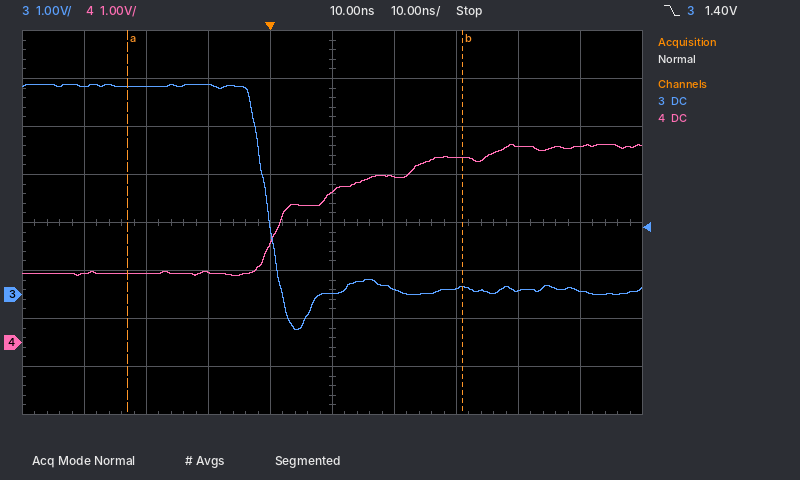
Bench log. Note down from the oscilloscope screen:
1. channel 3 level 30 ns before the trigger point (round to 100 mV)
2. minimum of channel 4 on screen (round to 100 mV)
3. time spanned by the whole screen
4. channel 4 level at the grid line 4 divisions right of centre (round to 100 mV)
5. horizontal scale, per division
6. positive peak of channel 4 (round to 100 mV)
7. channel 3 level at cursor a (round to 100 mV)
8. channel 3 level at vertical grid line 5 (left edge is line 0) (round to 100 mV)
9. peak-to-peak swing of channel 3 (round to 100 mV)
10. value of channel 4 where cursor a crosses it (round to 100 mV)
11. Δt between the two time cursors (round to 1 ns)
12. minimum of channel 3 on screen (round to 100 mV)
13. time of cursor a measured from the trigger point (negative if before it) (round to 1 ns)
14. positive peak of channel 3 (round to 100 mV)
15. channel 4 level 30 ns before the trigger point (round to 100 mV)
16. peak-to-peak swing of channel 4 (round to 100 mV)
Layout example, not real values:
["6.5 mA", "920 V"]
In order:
["4.3 V", "1.4 V", "100 ns", "4.1 V", "10 ns", "4.1 V", "4.3 V", "0.0 V", "5.1 V", "1.4 V", "54 ns", "-700 mV", "-23 ns", "4.4 V", "1.4 V", "2.7 V"]
